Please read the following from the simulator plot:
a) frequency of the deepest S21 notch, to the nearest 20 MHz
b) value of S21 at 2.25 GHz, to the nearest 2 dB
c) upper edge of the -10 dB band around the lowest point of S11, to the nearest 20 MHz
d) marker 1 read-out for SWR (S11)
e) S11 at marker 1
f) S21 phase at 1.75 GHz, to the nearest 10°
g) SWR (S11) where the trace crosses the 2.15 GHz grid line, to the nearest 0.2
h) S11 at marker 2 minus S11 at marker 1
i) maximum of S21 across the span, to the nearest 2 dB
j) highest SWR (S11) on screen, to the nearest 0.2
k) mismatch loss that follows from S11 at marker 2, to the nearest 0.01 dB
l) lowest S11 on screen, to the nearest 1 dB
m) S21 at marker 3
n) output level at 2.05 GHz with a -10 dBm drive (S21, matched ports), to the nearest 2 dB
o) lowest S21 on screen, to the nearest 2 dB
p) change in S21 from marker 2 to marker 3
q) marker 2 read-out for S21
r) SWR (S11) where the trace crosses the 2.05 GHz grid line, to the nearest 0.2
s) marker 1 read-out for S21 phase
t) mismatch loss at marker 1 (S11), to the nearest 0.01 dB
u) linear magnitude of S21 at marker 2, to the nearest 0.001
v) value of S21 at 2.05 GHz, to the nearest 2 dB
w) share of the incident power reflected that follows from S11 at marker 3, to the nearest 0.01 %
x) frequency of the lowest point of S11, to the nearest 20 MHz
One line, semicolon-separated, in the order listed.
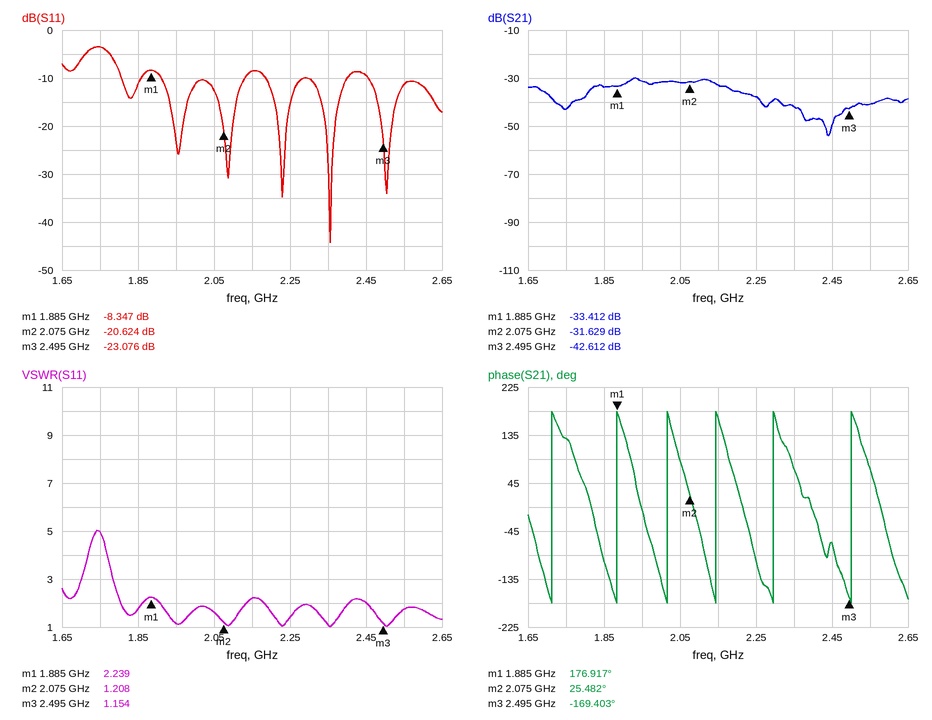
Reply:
2.44 GHz; -38 dB; 2.40 GHz; 2.239; -8.347 dB; 130°; 2.2; -12.277 dB; -30 dB; 5.0; 0.04 dB; -44 dB; -42.612 dB; -42 dBm; -54 dB; -10.983 dB; -31.629 dB; 1.6; 176.917°; 0.69 dB; 0.026; -32 dB; 0.49 %; 2.36 GHz
